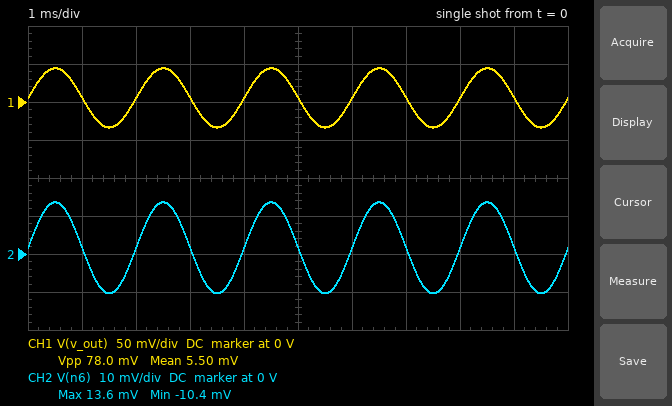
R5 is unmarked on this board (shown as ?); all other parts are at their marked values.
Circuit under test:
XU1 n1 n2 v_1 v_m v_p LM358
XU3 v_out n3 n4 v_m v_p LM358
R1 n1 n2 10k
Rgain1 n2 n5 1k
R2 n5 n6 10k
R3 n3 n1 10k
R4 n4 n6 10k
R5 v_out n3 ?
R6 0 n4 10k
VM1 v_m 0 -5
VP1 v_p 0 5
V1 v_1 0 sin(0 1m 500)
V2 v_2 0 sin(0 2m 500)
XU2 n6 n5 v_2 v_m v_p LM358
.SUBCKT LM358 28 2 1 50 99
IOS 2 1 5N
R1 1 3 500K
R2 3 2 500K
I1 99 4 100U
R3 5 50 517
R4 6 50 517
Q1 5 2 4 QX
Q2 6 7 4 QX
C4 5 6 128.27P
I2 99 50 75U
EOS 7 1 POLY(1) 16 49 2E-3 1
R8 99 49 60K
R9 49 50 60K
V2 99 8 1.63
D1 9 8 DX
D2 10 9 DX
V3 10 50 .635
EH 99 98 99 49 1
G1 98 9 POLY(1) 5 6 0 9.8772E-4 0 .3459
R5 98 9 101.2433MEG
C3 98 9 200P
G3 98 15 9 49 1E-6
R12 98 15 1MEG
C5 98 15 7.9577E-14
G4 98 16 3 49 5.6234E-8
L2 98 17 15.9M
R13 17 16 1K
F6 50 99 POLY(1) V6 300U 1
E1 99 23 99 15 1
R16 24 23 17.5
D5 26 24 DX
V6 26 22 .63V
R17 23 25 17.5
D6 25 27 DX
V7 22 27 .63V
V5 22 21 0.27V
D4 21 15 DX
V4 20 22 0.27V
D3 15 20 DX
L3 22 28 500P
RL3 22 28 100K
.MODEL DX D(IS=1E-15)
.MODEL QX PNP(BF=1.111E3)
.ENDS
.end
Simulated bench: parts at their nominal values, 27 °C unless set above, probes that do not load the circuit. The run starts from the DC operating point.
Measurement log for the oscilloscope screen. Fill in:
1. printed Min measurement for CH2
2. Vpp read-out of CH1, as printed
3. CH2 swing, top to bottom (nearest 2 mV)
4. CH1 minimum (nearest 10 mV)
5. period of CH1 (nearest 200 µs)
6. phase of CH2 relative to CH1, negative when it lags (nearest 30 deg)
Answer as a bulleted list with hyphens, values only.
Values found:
- -10.4 mV
- 78.0 mV
- 24 mV
- -30 mV
- 2.0 ms
- 0 deg
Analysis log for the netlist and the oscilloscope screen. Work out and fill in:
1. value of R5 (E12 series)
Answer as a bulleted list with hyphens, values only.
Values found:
- 22 kΩ
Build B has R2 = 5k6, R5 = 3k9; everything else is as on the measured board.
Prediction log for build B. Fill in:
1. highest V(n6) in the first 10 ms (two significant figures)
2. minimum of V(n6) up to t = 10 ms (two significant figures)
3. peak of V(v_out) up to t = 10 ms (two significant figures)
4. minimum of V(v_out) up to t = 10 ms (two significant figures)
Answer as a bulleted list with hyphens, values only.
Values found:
- 9.4 mV
- -5.8 mV
- 12 mV
- -5.2 mV
